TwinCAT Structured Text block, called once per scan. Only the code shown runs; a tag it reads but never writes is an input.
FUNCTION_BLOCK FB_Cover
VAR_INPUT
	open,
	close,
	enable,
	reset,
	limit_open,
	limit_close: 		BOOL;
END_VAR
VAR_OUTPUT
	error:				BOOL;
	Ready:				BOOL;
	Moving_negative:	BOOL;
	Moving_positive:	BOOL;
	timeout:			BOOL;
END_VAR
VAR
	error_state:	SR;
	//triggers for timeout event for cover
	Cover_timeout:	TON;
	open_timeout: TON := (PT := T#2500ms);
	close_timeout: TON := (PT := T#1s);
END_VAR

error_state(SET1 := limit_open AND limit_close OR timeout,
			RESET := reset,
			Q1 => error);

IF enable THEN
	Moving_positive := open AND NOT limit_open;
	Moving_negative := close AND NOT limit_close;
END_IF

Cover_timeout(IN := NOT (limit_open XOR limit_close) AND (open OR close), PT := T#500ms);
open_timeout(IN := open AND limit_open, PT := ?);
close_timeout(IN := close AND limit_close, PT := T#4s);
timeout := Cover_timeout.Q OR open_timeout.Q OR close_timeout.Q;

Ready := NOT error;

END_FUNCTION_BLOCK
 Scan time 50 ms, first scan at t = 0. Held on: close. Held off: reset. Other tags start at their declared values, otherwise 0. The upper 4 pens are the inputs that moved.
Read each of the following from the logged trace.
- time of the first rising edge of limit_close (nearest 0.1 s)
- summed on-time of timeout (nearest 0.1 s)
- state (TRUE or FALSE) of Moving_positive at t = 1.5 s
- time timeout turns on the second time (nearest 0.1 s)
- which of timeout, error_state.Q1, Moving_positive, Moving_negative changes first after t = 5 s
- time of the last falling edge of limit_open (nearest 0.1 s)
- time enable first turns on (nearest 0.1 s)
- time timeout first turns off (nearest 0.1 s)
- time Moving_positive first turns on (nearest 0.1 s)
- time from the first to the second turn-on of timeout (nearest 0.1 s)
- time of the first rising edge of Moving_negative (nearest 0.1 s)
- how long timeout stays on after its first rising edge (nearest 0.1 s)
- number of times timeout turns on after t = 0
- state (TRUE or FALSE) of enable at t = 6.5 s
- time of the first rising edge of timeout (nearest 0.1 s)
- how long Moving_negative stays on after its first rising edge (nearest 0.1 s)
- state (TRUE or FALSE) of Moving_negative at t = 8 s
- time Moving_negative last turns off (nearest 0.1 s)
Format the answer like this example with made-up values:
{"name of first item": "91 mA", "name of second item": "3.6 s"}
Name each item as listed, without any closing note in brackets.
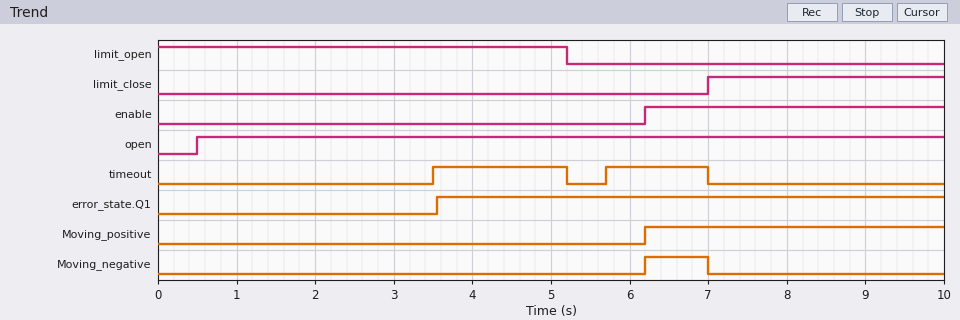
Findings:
{"time of the first rising edge of limit_close": "7.0 s", "summed on-time of timeout": "3.0 s", "state (TRUE or FALSE) of Moving_positive at t = 1.5 s": "FALSE", "time timeout turns on the second time": "5.7 s", "which of timeout, error_state.Q1, Moving_positive, Moving_negative changes first after t = 5 s": "timeout", "time of the last falling edge of limit_open": "5.2 s", "time enable first turns on": "6.2 s", "time timeout first turns off": "5.2 s", "time Moving_positive first turns on": "6.2 s", "time from the first to the second turn-on of timeout": "2.2 s", "time of the first rising edge of Moving_negative": "6.2 s", "how long timeout stays on after its first rising edge": "1.7 s", "number of times timeout turns on after t = 0": "2", "state (TRUE or FALSE) of enable at t = 6.5 s": "TRUE", "time of the first rising edge of timeout": "3.5 s", "how long Moving_negative stays on after its first rising edge": "0.8 s", "state (TRUE or FALSE) of Moving_negative at t = 8 s": "FALSE", "time Moving_negative last turns off": "7.0 s"}
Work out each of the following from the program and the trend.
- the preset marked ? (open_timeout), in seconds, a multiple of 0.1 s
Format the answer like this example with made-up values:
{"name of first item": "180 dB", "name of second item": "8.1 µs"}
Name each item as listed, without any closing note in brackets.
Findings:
{"the preset marked ? (open_timeout), in seconds, a multiple of 0.1 s": "3.0 s"}
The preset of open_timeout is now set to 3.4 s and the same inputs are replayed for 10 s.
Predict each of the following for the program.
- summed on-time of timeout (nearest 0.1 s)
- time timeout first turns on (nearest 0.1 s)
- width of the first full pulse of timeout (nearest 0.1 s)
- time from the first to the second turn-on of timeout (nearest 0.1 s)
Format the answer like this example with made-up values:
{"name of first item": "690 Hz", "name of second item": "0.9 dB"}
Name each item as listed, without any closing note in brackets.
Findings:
{"summed on-time of timeout": "2.6 s", "time timeout first turns on": "3.9 s", "width of the first full pulse of timeout": "1.3 s", "time from the first to the second turn-on of timeout": "1.8 s"}
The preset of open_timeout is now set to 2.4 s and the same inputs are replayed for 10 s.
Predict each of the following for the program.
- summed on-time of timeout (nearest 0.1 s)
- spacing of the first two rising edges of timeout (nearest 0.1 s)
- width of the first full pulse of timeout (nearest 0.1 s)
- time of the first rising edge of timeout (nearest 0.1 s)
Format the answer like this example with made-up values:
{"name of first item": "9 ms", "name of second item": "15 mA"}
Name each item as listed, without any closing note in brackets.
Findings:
{"summed on-time of timeout": "3.6 s", "spacing of the first two rising edges of timeout": "2.8 s", "width of the first full pulse of timeout": "2.3 s", "time of the first rising edge of timeout": "2.9 s"}
